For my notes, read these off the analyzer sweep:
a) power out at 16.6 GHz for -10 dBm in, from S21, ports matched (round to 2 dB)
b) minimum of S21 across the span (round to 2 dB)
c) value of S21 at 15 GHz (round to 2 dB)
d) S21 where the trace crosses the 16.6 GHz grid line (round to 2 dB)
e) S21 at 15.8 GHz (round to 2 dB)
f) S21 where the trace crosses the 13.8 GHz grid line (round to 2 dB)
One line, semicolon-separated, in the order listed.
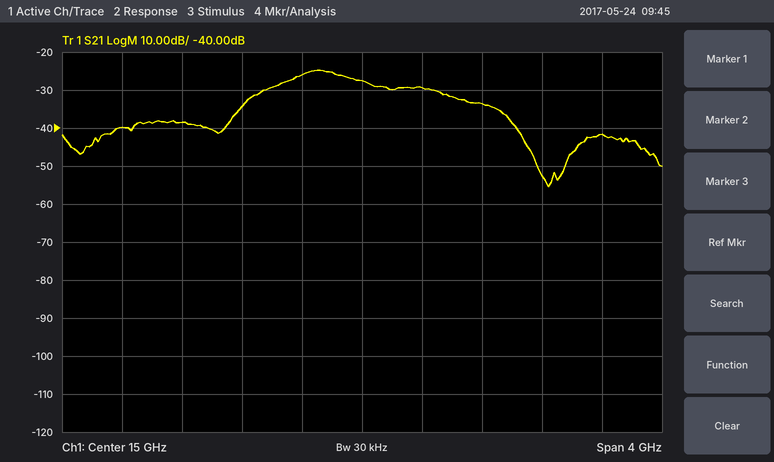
-52 dBm; -56 dB; -28 dB; -42 dB; -34 dB; -38 dB
